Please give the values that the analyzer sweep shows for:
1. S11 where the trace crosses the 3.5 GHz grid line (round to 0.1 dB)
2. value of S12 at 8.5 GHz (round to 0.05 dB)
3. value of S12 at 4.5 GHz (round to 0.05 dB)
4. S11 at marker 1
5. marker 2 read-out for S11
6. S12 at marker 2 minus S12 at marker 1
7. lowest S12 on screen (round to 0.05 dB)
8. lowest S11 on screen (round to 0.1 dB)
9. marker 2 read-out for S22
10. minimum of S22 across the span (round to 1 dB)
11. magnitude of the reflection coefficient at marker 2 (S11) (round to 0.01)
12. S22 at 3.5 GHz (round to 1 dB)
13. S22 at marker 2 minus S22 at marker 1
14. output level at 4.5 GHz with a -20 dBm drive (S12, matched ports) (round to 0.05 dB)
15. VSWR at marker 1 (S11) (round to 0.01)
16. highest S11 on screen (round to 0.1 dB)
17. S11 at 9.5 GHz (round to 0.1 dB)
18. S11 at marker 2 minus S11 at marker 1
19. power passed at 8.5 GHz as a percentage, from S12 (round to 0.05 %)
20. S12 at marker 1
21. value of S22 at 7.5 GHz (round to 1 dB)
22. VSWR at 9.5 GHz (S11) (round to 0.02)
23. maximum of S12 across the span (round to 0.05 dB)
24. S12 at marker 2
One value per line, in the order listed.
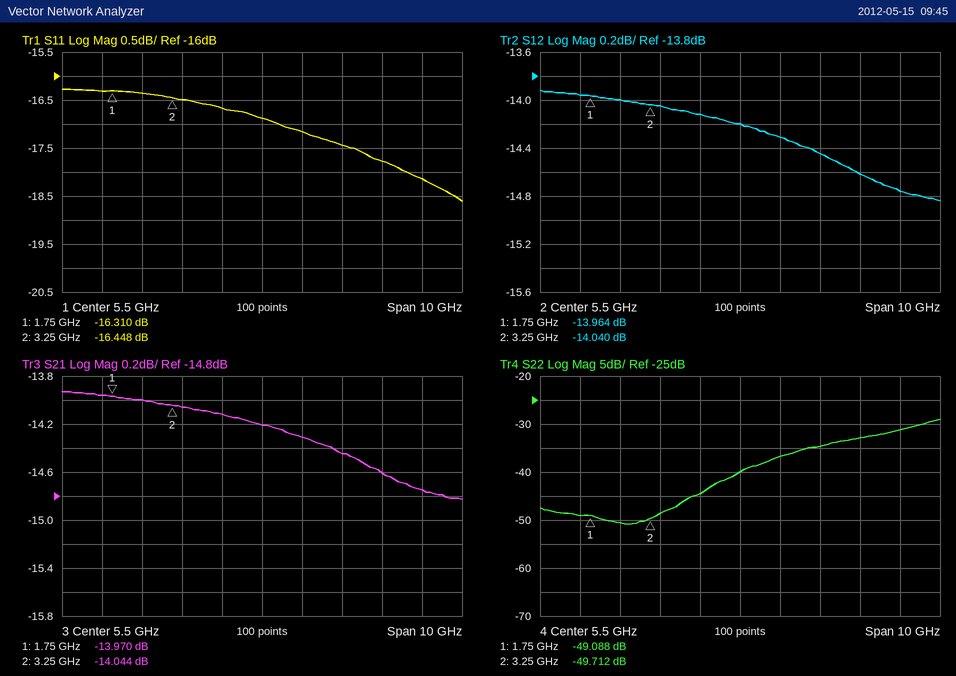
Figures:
-16.5 dB
-14.60 dB
-14.10 dB
-16.310 dB
-16.448 dB
-0.076 dB
-14.85 dB
-18.6 dB
-49.712 dB
-51 dB
0.15
-49 dB
-0.624 dB
-34.10 dBm
1.36
-16.3 dB
-18.1 dB
-0.138 dB
3.45 %
-13.964 dB
-35 dB
1.28
-13.90 dB
-14.040 dB
